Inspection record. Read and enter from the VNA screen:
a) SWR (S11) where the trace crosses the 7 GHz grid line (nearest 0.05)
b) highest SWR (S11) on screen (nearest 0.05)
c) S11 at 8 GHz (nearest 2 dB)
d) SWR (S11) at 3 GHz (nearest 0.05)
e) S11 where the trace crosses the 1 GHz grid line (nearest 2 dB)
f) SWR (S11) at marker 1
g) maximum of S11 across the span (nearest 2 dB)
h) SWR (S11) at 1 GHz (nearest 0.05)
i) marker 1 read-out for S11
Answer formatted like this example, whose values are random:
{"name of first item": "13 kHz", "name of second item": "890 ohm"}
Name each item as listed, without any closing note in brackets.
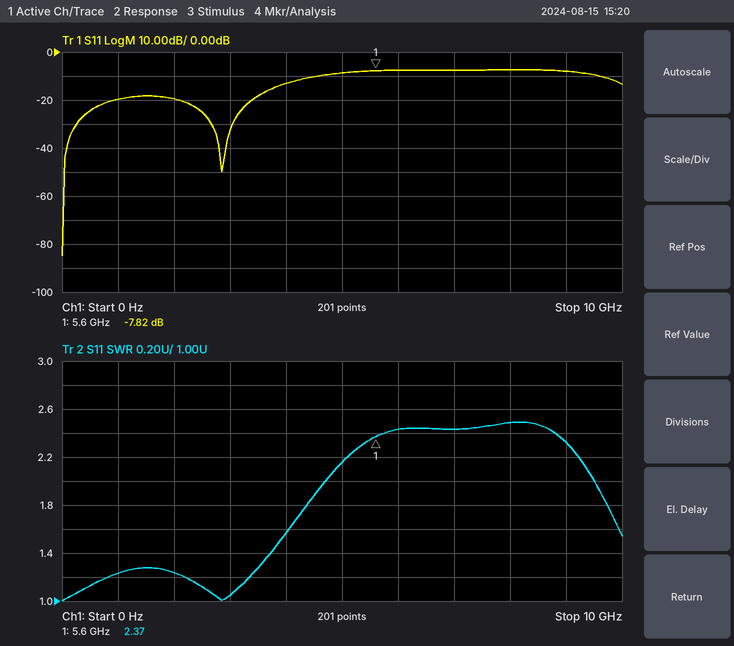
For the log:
{"SWR (S11) where the trace crosses the 7 GHz grid line": "2.45", "highest SWR (S11) on screen": "2.50", "S11 at 8 GHz": "-8 dB", "SWR (S11) at 3 GHz": "1.05", "S11 where the trace crosses the 1 GHz grid line": "-20 dB", "SWR (S11) at marker 1": "2.37", "maximum of S11 across the span": "-8 dB", "SWR (S11) at 1 GHz": "1.25", "marker 1 read-out for S11": "-7.82 dB"}
